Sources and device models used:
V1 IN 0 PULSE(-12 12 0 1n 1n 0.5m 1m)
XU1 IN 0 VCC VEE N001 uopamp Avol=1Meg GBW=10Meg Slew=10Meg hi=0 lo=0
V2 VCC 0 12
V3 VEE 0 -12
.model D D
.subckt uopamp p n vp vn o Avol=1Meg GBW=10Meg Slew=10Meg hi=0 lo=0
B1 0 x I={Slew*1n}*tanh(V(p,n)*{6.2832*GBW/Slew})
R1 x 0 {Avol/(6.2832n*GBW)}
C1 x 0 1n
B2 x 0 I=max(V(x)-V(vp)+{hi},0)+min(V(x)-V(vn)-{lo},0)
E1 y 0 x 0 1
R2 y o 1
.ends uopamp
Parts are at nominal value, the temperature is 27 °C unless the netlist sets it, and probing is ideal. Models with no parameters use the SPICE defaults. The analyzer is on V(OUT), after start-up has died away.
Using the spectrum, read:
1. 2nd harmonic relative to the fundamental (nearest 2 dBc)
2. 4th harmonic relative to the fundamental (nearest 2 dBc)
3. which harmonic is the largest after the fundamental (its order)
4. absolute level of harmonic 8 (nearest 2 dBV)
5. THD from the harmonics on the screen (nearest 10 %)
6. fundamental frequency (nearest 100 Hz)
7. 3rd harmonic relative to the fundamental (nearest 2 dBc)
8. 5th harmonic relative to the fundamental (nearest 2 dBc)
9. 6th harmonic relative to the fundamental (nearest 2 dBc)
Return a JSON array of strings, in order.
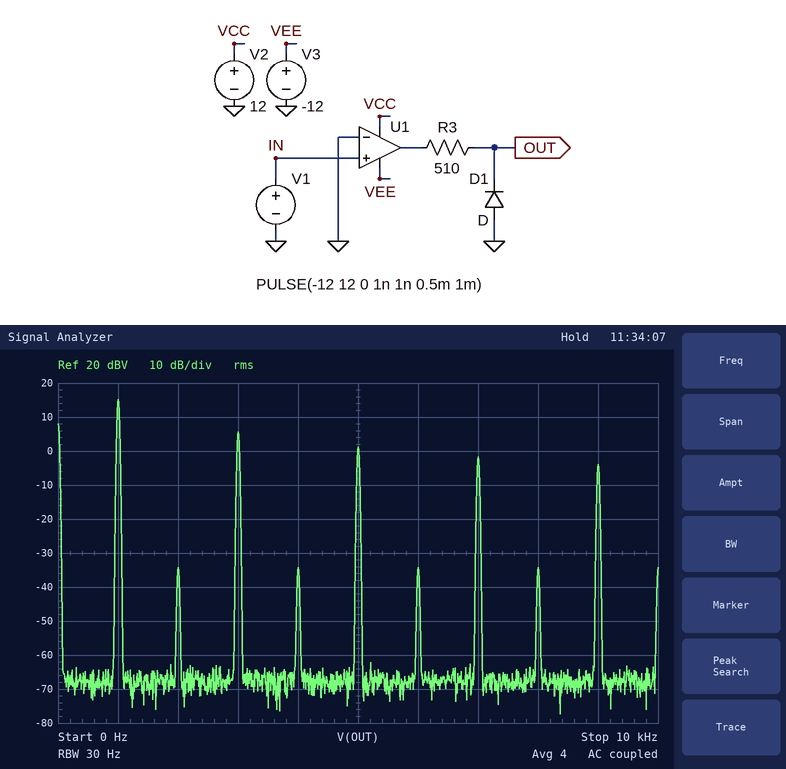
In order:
["-50 dBc", "-50 dBc", "3", "-34 dBV", "40 %", "1.0 kHz", "-10 dBc", "-14 dBc", "-50 dBc"]
